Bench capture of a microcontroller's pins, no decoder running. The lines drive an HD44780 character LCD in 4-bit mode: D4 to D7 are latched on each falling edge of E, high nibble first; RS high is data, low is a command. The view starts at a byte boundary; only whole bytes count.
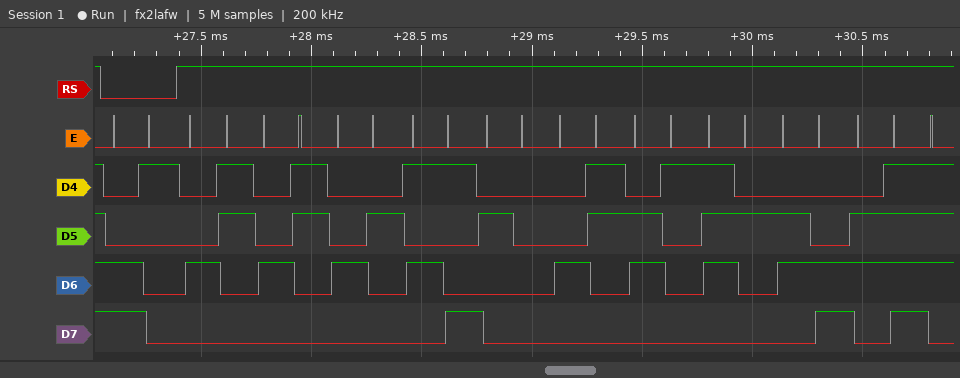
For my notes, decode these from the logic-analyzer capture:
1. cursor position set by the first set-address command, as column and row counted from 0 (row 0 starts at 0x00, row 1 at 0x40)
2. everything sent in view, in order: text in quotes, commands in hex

column 1, row 1
0xC1 "CCBY Carlo"
